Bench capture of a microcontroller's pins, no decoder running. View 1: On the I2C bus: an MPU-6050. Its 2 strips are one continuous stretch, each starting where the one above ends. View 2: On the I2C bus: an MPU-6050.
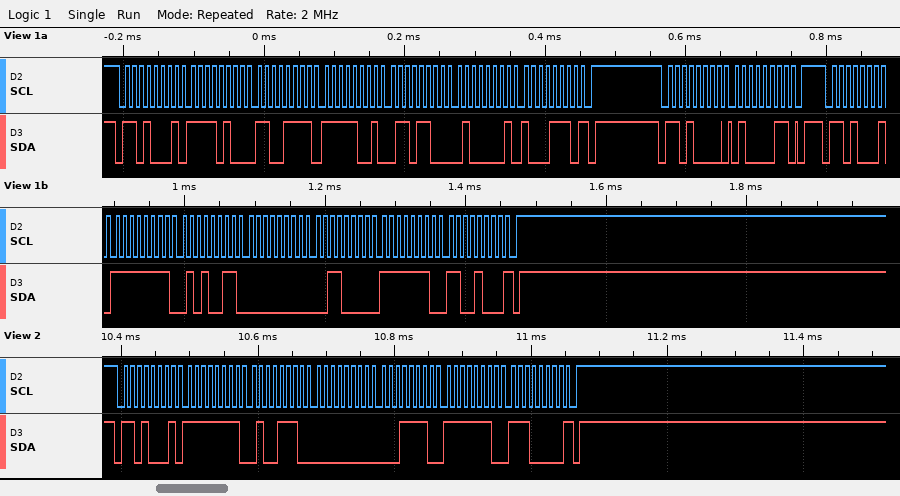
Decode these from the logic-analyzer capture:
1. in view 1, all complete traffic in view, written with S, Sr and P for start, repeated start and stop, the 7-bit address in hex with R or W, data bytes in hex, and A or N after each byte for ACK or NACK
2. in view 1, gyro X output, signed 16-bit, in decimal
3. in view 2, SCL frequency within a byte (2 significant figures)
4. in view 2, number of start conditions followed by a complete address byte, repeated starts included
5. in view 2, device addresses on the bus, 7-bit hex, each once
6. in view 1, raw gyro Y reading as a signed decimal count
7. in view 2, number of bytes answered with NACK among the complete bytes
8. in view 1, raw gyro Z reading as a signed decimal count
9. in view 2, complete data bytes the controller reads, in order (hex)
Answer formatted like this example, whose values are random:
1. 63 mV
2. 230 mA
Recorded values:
1. S 68R A F4 A CF A F9 A 6C A 41 A 8E N P S 68W A 43 A P S 68R A FF A 53 A 00 A 30 A FE A C8 N P
2. -173
3. 100 kHz
4. 1
5. 0x68
6. 48
7. 1
8. -312
9. FF 4E 00 1E FE E0
